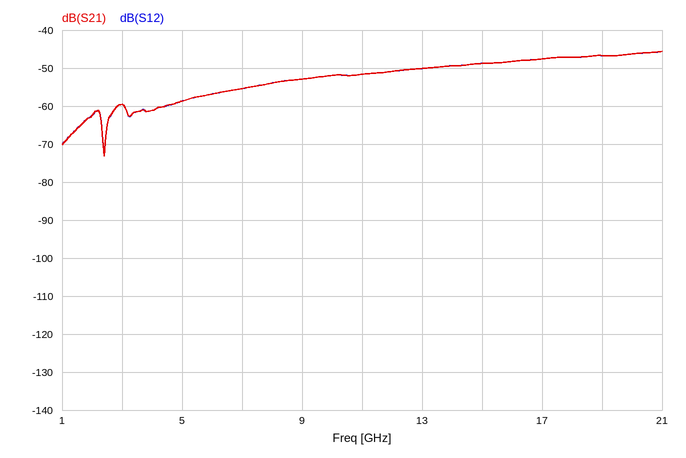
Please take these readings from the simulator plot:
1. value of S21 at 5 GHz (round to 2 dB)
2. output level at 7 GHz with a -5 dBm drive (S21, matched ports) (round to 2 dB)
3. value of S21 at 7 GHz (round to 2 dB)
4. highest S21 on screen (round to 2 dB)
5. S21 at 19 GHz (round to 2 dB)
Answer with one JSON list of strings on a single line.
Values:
["-58 dB", "-60 dBm", "-56 dB", "-46 dB", "-46 dB"]
